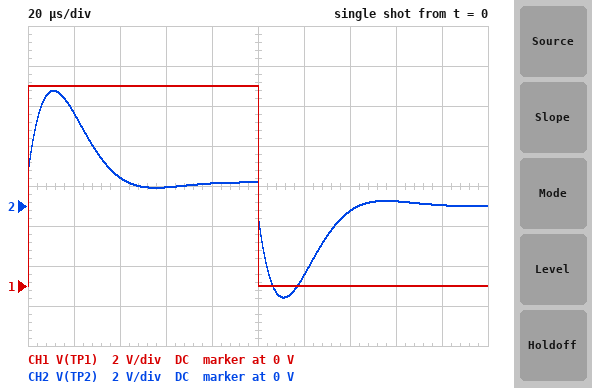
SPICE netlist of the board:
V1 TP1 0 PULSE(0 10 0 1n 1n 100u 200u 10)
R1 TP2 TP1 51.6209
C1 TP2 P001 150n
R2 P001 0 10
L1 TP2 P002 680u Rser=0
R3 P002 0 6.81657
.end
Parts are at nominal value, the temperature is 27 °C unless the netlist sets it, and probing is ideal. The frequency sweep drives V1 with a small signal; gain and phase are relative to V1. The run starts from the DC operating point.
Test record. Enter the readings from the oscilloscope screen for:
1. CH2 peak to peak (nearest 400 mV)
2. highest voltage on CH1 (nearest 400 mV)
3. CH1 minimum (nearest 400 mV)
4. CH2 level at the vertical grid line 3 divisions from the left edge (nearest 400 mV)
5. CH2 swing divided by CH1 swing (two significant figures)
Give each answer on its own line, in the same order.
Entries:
10.4 V
10.0 V
0 V
800 mV
1.0
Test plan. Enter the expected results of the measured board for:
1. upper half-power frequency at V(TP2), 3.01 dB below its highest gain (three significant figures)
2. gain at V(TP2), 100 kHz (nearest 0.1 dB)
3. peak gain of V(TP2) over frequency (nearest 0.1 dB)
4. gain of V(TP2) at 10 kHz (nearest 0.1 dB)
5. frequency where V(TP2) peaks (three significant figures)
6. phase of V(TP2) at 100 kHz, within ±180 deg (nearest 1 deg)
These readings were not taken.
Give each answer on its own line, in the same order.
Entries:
29.7 kHz
-12.5 dB
-1.5 dB
-3.0 dB
15.4 kHz
-36 deg
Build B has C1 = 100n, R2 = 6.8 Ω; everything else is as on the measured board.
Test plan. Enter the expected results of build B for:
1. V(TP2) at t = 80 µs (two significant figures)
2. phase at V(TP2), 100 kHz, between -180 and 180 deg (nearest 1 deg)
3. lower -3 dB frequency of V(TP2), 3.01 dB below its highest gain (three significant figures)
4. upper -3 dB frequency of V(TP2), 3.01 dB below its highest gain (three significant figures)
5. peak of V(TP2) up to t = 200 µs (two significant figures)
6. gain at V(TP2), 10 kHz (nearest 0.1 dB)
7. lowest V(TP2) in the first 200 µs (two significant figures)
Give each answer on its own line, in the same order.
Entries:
1.2 V
-50 deg
9.30 kHz
40.1 kHz
6.5 V
-3.4 dB
-5.3 V
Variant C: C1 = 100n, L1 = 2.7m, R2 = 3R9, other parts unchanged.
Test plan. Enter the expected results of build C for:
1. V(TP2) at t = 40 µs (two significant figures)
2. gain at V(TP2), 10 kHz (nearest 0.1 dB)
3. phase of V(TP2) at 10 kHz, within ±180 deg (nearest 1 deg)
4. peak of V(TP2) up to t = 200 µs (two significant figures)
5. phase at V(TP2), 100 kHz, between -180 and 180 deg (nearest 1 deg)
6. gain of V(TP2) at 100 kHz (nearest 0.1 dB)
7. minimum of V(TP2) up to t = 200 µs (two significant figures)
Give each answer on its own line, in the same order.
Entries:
5.6 V
-0.2 dB
-1 deg
8.3 V
-60 deg
-10.9 dB
-6.4 V
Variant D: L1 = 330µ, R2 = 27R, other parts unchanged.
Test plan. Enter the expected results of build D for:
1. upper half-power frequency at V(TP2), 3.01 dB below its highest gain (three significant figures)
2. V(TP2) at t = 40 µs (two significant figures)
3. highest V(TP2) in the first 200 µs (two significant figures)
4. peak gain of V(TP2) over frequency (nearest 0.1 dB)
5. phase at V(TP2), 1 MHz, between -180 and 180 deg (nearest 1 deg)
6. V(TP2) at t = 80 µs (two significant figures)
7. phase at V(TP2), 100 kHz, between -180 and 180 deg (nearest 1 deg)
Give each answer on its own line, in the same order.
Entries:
54.4 kHz
950 mV
4.3 V
-4.3 dB
-1 deg
1.2 V
-9 deg
